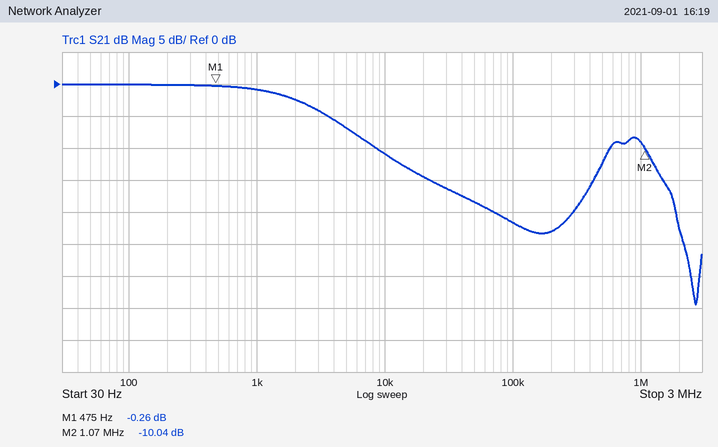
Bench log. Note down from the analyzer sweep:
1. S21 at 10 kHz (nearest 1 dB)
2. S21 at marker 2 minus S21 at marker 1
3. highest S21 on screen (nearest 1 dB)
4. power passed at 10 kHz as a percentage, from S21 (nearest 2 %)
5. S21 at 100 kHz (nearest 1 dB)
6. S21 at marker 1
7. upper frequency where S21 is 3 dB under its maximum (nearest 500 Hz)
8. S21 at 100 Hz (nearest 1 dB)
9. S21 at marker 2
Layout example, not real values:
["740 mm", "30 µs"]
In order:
["-11 dB", "-9.78 dB", "0 dB", "8 %", "-22 dB", "-0.26 dB", "2.5 kHz", "0 dB", "-10.04 dB"]
